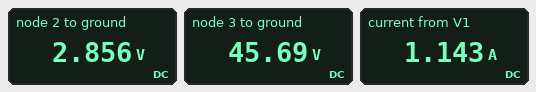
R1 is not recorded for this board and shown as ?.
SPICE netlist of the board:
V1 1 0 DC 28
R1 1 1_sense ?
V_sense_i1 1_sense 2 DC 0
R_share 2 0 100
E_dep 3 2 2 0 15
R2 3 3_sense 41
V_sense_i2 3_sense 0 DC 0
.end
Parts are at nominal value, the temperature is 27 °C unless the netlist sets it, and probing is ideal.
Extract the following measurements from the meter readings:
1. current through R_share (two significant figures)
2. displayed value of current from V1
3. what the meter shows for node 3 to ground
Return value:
29 mA
1.143 A
45.69 V
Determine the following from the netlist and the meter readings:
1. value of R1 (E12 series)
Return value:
22 Ω
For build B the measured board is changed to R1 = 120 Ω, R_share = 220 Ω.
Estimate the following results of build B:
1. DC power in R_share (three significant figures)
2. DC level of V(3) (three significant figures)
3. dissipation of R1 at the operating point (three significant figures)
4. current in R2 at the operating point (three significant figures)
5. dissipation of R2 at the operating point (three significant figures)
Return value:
1.52 mW
9.26 V
6.27 W
226 mA
2.09 W
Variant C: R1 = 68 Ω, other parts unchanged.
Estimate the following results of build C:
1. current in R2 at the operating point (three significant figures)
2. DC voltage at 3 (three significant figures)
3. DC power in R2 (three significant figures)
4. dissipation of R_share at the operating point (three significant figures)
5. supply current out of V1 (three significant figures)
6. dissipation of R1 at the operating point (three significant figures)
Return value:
387 mA
15.9 V
6.15 W
9.85 mW
397 mA
10.7 W
